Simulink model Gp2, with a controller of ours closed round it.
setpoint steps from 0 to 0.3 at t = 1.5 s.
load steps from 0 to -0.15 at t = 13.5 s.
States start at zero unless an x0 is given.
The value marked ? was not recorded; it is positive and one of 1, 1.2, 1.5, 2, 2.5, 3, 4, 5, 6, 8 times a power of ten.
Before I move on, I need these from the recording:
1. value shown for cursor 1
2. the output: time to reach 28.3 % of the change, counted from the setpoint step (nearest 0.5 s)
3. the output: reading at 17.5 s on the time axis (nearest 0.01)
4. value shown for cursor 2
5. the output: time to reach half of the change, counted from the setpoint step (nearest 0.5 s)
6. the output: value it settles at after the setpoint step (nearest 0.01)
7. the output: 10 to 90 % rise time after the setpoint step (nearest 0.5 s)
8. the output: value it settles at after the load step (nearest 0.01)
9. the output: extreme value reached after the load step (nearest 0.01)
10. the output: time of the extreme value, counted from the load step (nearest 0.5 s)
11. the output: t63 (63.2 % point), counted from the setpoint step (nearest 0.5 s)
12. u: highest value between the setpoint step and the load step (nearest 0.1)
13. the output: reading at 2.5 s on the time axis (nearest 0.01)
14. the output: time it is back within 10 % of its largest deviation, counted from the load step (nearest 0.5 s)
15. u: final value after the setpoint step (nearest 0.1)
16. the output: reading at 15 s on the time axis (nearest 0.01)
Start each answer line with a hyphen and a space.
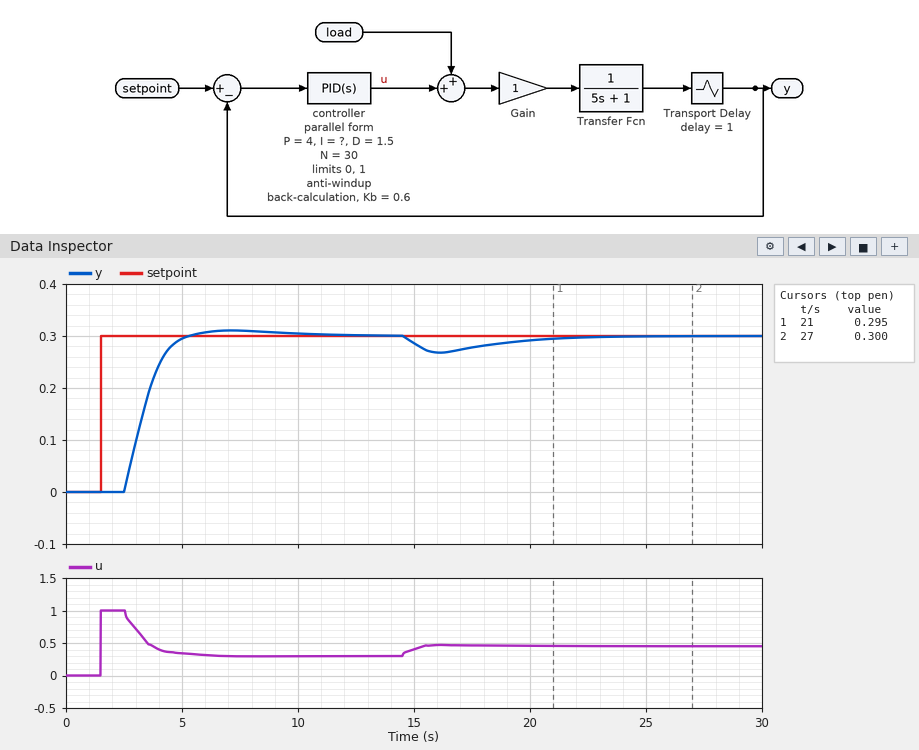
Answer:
- 0.295
- 1.5 s
- 0.28
- 0.300
- 2.0 s
- 0.30
- 1.5 s
- 0.30
- 0.27
- 2.5 s
- 2.0 s
- 1.0
- 0.00
- 8.5 s
- 0.3
- 0.29
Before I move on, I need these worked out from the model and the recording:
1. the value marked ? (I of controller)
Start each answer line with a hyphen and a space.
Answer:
- 1.2
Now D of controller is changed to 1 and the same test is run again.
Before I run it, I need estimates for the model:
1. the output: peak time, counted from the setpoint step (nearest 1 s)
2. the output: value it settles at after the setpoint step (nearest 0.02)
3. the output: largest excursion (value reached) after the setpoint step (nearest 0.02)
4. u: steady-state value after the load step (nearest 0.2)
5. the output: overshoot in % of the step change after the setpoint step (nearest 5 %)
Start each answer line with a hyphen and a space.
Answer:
- 4 s
- 0.30
- 0.32
- 0.4
- 10 %
